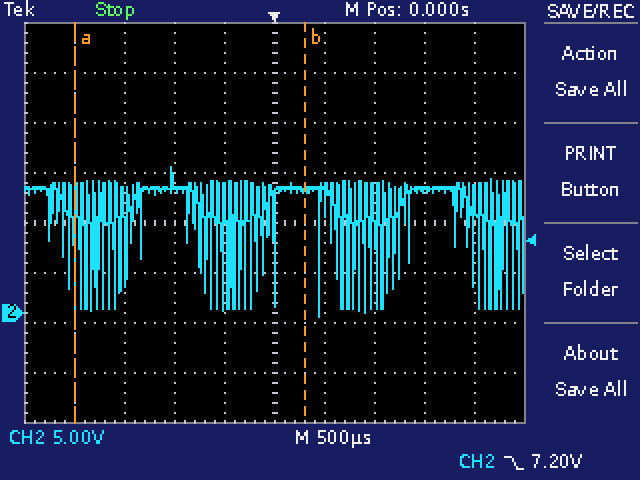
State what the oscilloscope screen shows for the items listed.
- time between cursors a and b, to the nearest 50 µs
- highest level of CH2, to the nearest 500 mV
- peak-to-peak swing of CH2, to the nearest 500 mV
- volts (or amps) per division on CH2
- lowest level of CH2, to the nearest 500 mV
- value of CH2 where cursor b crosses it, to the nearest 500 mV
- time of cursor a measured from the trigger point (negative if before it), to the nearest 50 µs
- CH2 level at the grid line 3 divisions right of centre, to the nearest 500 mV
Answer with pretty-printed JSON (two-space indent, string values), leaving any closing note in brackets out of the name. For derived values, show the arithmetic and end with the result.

{
  "time between cursors a and b, to the nearest 50 µs": "2.30 ms",
  "highest level of CH2, to the nearest 500 mV": "14.5 V",
  "peak-to-peak swing of CH2, to the nearest 500 mV": "14.5 V − (-500 mV) = 15.0 V",
  "volts (or amps) per division on CH2": "5 V",
  "lowest level of CH2, to the nearest 500 mV": "-500 mV",
  "value of CH2 where cursor b crosses it, to the nearest 500 mV": "12.5 V",
  "time of cursor a measured from the trigger point (negative if before it), to the nearest 50 µs": "-2.00 ms",
  "CH2 level at the grid line 3 divisions right of centre, to the nearest 500 mV": "12.5 V"
}
